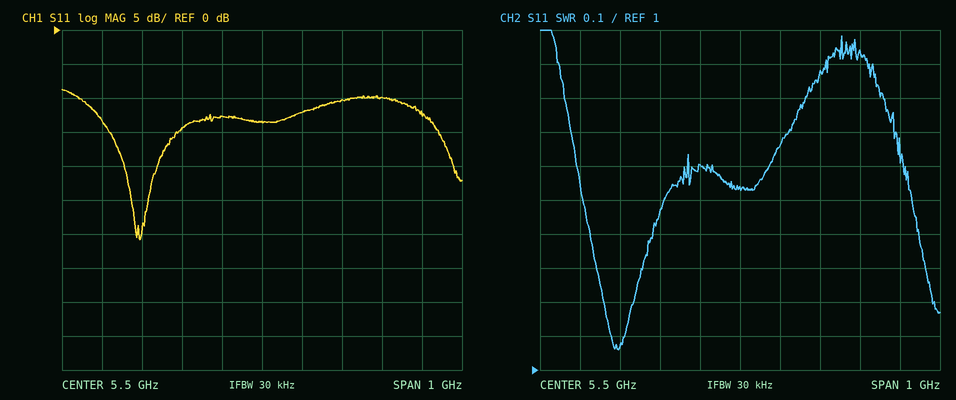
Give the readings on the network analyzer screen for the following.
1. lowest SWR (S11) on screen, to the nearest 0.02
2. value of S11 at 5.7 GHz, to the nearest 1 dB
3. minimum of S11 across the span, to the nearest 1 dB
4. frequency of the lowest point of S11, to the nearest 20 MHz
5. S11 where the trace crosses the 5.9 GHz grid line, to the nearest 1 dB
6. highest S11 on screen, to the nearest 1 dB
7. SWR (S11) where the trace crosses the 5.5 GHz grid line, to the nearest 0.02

1.06
-10 dB
-31 dB
5.20 GHz
-12 dB
-9 dB
1.54
